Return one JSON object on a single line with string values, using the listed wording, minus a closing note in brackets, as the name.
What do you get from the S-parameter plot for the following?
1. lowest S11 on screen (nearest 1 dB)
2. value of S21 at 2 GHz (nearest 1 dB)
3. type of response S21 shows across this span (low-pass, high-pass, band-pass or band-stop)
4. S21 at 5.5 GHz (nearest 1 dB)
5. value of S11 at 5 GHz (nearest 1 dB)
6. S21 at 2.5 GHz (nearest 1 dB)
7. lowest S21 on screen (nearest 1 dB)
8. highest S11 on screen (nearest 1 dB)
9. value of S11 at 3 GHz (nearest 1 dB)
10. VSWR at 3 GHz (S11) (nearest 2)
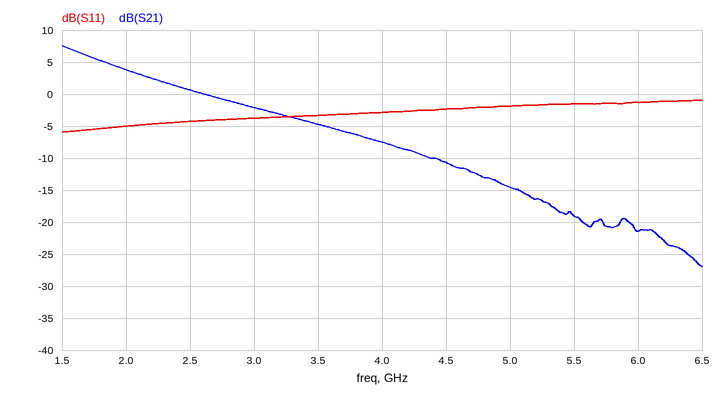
{"lowest S11 on screen": "-6 dB", "value of S21 at 2 GHz": "4 dB", "type of response S21 shows across this span": "low-pass", "S21 at 5.5 GHz": "-19 dB", "value of S11 at 5 GHz": "-2 dB", "S21 at 2.5 GHz": "1 dB", "lowest S21 on screen": "-27 dB", "highest S11 on screen": "-1 dB", "value of S11 at 3 GHz": "-4 dB", "VSWR at 3 GHz (S11)": "4"}
